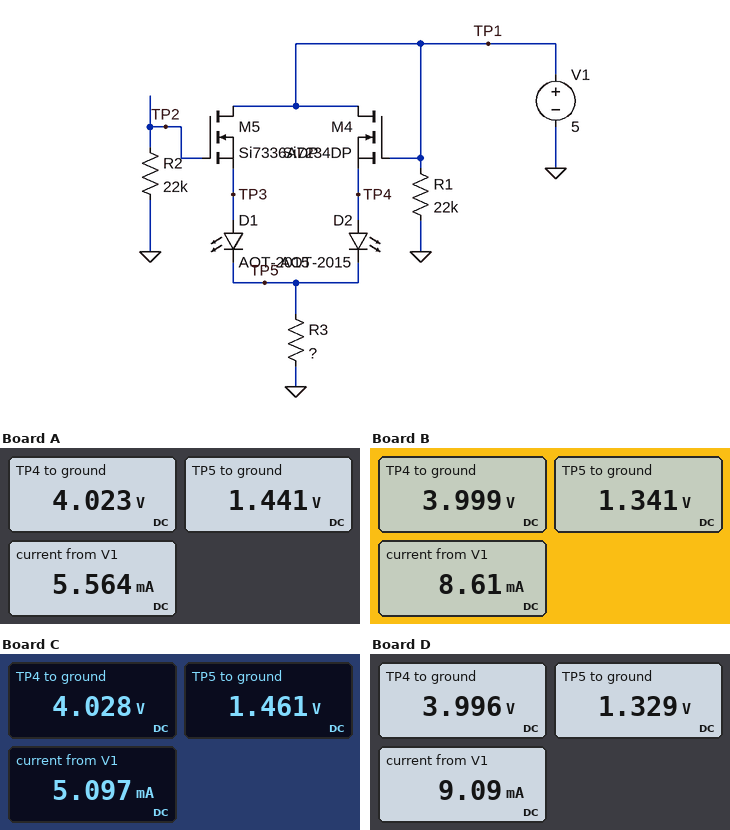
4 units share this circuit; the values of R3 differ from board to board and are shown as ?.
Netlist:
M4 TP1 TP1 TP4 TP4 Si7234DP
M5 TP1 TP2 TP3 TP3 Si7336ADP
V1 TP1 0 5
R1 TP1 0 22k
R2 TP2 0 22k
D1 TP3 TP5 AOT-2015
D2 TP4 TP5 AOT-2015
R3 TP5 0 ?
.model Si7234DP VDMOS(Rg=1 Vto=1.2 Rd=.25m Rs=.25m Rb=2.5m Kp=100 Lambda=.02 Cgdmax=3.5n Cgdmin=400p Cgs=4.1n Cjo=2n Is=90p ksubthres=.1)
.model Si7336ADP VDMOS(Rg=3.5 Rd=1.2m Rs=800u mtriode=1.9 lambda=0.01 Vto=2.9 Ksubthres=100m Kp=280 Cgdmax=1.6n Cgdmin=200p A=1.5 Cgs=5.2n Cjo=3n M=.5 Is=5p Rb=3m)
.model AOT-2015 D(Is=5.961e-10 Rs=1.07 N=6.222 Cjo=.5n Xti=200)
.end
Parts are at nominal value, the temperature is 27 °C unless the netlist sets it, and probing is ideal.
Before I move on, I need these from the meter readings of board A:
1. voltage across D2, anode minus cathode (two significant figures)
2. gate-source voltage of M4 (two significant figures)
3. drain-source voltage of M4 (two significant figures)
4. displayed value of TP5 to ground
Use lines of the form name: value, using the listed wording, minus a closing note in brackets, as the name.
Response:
voltage across D2, anode minus cathode: 2.6 V
gate-source voltage of M4: 980 mV
drain-source voltage of M4: 980 mV
displayed value of TP5 to ground: 1.441 V
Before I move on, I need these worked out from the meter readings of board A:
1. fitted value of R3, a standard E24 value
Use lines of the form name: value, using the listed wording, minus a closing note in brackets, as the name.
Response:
fitted value of R3, a standard E24 value: 270 Ω
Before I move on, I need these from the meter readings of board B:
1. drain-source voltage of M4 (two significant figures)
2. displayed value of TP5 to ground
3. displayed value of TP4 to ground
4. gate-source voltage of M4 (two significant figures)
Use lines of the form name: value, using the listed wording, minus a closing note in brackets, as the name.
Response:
drain-source voltage of M4: 1.0 V
displayed value of TP5 to ground: 1.341 V
displayed value of TP4 to ground: 3.999 V
gate-source voltage of M4: 1.0 V
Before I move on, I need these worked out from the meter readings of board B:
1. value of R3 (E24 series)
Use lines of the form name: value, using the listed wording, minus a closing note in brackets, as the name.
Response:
value of R3: 160 Ω
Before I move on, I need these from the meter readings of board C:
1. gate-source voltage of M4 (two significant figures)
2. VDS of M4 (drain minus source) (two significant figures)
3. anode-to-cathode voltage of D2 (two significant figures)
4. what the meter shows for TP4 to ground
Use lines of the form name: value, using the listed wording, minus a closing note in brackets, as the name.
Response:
gate-source voltage of M4: 970 mV
VDS of M4 (drain minus source): 970 mV
anode-to-cathode voltage of D2: 2.6 V
what the meter shows for TP4 to ground: 4.028 V
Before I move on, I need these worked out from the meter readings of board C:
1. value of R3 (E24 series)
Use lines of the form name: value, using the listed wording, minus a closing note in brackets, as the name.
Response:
value of R3: 300 Ω
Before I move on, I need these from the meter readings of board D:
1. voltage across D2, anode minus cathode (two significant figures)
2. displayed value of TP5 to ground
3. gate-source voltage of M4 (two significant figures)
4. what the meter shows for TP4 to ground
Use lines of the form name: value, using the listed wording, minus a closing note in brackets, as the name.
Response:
voltage across D2, anode minus cathode: 2.7 V
displayed value of TP5 to ground: 1.329 V
gate-source voltage of M4: 1.0 V
what the meter shows for TP4 to ground: 3.996 V
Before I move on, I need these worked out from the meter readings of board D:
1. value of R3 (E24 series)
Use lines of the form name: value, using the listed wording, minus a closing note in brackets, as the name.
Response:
value of R3: 150 Ω
